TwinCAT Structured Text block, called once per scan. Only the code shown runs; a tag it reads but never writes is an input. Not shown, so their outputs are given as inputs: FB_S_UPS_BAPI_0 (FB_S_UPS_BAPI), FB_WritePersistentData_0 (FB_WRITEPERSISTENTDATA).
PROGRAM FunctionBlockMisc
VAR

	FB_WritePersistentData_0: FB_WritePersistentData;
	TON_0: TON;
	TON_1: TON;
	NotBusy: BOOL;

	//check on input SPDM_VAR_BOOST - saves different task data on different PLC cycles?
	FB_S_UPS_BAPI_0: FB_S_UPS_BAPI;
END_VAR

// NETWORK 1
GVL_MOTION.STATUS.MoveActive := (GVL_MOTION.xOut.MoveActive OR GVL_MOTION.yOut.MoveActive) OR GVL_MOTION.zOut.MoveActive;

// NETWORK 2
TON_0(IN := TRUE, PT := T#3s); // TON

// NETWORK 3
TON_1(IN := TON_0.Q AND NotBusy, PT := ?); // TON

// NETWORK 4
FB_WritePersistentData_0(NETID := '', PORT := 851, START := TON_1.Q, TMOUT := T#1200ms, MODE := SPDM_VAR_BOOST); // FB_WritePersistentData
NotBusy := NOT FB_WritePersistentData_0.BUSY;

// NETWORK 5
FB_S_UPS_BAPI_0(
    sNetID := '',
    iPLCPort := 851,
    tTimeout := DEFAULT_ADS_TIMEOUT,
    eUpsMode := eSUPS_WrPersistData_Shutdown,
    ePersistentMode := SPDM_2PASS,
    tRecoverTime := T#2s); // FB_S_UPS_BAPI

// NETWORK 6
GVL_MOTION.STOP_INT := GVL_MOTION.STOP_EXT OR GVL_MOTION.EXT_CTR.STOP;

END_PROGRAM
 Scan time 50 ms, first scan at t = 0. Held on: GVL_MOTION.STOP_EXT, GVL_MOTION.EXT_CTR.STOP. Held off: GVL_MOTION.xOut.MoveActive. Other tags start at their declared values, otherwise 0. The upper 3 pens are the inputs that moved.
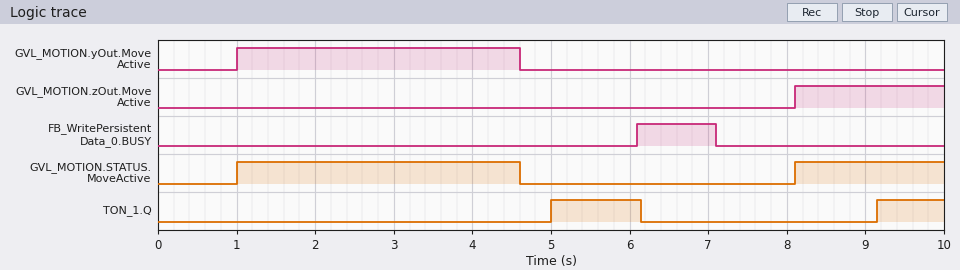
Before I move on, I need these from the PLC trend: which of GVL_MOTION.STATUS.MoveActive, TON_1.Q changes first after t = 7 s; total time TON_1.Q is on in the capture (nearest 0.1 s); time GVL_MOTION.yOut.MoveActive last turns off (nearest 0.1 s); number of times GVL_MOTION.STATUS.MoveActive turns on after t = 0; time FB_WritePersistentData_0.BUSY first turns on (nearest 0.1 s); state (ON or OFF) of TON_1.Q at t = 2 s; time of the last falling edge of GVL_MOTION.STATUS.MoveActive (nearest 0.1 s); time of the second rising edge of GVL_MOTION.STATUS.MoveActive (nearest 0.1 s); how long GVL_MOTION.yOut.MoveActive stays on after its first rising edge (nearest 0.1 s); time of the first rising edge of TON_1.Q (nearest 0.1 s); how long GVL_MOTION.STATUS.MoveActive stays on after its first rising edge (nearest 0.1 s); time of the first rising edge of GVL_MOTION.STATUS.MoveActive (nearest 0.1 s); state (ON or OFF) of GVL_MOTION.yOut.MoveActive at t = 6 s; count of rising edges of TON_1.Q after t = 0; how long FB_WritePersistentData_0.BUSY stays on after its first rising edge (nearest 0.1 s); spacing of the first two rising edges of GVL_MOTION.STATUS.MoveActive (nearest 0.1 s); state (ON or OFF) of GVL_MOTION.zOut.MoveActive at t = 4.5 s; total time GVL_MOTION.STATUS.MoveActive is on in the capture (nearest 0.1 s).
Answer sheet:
GVL_MOTION.STATUS.MoveActive
2.0 s
4.6 s
2
6.1 s
OFF
4.6 s
8.1 s
3.6 s
5.0 s
3.6 s
1.0 s
OFF
2
1.0 s
7.1 s
OFF
5.5 s
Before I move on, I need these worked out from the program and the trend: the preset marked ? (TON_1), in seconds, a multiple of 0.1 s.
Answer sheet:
2.0 s
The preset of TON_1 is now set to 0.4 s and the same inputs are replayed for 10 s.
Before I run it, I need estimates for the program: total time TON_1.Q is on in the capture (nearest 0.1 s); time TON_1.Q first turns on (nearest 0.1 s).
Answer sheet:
5.2 s
3.4 s
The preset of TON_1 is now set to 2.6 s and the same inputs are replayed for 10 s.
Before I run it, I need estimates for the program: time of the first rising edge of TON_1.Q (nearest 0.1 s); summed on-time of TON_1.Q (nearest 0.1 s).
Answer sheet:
5.6 s
0.8 s
